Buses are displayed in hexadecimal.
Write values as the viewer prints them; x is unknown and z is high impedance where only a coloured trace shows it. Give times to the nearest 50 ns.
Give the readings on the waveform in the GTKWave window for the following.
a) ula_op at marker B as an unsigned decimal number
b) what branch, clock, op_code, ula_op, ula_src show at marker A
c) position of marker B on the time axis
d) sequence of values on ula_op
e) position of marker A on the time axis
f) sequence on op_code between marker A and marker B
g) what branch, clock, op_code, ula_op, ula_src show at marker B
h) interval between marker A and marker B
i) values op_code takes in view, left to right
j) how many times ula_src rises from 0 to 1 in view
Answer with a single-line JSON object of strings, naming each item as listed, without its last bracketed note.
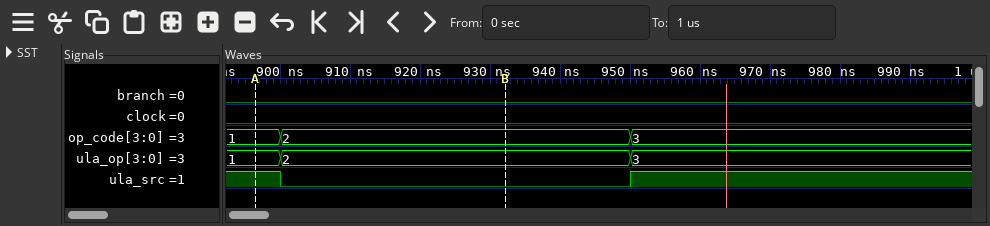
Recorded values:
{"ula_op at marker B as an unsigned decimal number": "2", "what branch, clock, op_code, ula_op, ula_src show at marker A": "branch=0, clock=0, op_code=1, ula_op=1, ula_src=1", "position of marker B on the time axis": "950 ns", "sequence of values on ula_op": "1, 2, 3", "position of marker A on the time axis": "900 ns", "sequence on op_code between marker A and marker B": "1, 2", "what branch, clock, op_code, ula_op, ula_src show at marker B": "branch=0, clock=0, op_code=2, ula_op=2, ula_src=0", "interval between marker A and marker B": "50 ns", "values op_code takes in view, left to right": "1, 2, 3", "how many times ula_src rises from 0 to 1 in view": "1"}
